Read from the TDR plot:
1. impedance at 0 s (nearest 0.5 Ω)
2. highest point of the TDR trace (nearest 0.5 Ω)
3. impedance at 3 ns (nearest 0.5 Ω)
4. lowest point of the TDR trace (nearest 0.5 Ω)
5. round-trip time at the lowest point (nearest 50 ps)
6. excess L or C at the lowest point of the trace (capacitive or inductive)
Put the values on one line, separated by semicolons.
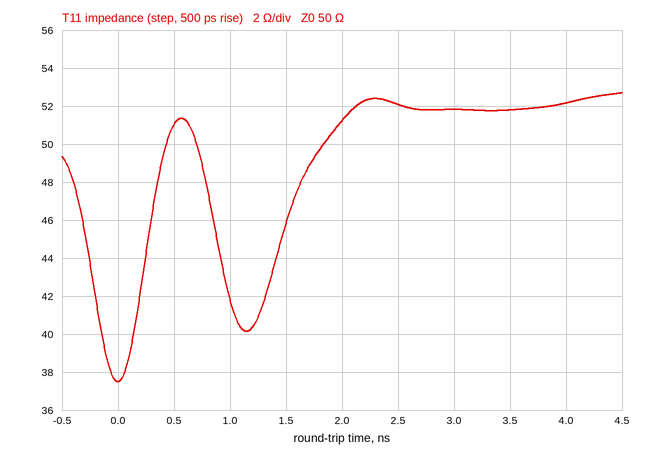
37.5 Ω; 52.5 Ω; 52.0 Ω; 37.5 Ω; 0 ps; capacitive
